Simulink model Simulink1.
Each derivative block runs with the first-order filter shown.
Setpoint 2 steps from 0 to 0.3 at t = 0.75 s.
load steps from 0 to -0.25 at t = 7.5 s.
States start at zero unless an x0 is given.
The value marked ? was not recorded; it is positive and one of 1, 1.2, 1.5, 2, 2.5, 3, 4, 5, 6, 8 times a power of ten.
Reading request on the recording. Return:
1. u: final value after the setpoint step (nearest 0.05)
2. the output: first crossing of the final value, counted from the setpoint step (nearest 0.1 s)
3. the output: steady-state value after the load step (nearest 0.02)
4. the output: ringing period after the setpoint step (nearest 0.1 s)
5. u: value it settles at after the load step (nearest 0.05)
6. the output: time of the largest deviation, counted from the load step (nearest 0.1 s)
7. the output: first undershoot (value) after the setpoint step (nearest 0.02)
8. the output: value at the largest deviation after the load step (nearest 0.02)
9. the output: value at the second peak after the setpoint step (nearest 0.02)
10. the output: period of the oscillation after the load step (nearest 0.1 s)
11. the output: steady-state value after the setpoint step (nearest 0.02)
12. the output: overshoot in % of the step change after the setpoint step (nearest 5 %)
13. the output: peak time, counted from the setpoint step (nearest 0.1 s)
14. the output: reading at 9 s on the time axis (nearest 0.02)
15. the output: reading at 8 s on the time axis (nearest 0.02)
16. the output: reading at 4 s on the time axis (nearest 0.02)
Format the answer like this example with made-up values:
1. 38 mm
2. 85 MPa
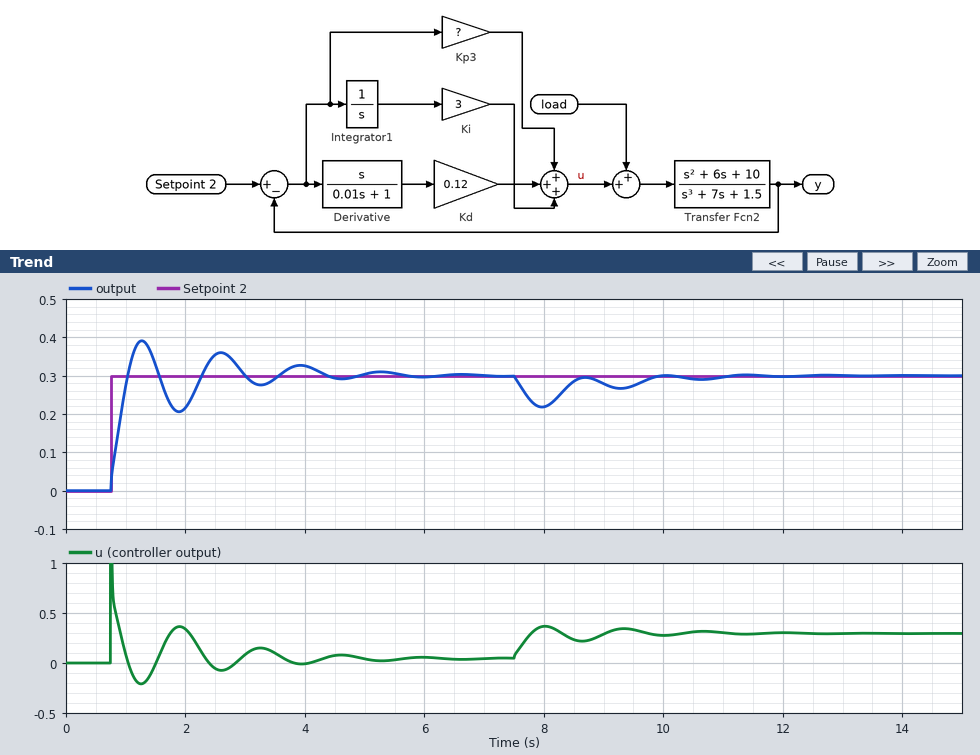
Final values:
1. 0.05
2. 0.3 s
3. 0.30
4. 1.3 s
5. 0.30
6. 0.5 s
7. 0.20
8. 0.22
9. 0.36
10. 1.3 s
11. 0.30
12. 30 %
13. 0.5 s
14. 0.28
15. 0.22
16. 0.32
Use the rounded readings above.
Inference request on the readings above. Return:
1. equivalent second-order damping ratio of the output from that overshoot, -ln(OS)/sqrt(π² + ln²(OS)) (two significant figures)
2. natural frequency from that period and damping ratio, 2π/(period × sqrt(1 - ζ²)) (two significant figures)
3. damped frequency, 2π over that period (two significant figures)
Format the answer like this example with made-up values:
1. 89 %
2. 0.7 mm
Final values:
1. 0.36
2. 5.2 rad/s
3. 4.8 rad/s
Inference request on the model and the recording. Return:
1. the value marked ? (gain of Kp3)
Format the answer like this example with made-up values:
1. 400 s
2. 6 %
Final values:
1. 3
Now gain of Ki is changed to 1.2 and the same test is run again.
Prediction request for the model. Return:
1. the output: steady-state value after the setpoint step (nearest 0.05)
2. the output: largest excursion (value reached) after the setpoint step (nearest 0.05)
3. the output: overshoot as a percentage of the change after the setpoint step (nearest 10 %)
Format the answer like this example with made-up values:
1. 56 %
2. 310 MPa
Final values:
1. 0.30
2. 0.35
3. 20 %
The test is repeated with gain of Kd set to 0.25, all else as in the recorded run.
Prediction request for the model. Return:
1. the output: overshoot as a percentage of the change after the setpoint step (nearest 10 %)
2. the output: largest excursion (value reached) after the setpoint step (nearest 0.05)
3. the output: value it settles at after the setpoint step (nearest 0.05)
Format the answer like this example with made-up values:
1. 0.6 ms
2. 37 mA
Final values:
1. 20 %
2. 0.35
3. 0.30
